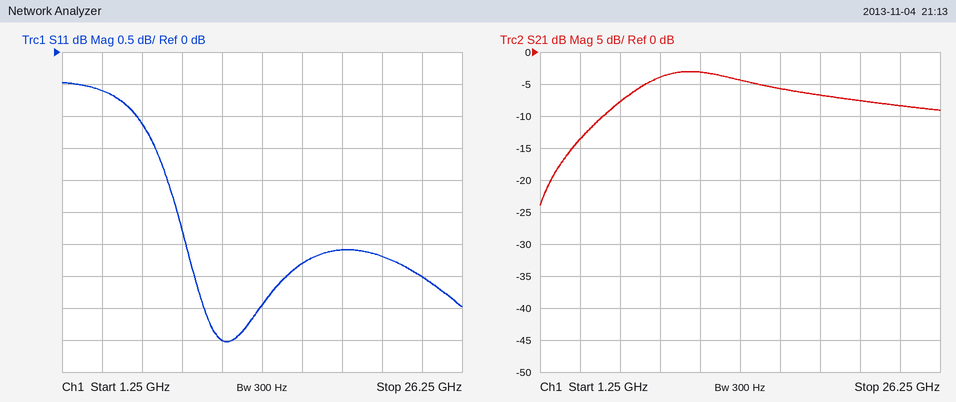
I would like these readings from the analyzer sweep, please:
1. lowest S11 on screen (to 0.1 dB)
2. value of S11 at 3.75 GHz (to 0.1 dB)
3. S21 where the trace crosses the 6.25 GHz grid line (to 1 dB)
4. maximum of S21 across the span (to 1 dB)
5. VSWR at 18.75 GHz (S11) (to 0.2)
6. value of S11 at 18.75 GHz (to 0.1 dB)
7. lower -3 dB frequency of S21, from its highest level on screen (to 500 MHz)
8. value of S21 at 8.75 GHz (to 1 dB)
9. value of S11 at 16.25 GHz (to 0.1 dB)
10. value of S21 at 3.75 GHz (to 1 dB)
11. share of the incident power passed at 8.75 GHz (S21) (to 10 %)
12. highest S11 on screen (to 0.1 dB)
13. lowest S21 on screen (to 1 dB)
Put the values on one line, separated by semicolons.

-4.5 dB; -0.6 dB; -8 dB; -3 dB; 5.6; -3.1 dB; 7.0 GHz; -4 dB; -3.3 dB; -14 dB; 40 %; -0.5 dB; -24 dB
